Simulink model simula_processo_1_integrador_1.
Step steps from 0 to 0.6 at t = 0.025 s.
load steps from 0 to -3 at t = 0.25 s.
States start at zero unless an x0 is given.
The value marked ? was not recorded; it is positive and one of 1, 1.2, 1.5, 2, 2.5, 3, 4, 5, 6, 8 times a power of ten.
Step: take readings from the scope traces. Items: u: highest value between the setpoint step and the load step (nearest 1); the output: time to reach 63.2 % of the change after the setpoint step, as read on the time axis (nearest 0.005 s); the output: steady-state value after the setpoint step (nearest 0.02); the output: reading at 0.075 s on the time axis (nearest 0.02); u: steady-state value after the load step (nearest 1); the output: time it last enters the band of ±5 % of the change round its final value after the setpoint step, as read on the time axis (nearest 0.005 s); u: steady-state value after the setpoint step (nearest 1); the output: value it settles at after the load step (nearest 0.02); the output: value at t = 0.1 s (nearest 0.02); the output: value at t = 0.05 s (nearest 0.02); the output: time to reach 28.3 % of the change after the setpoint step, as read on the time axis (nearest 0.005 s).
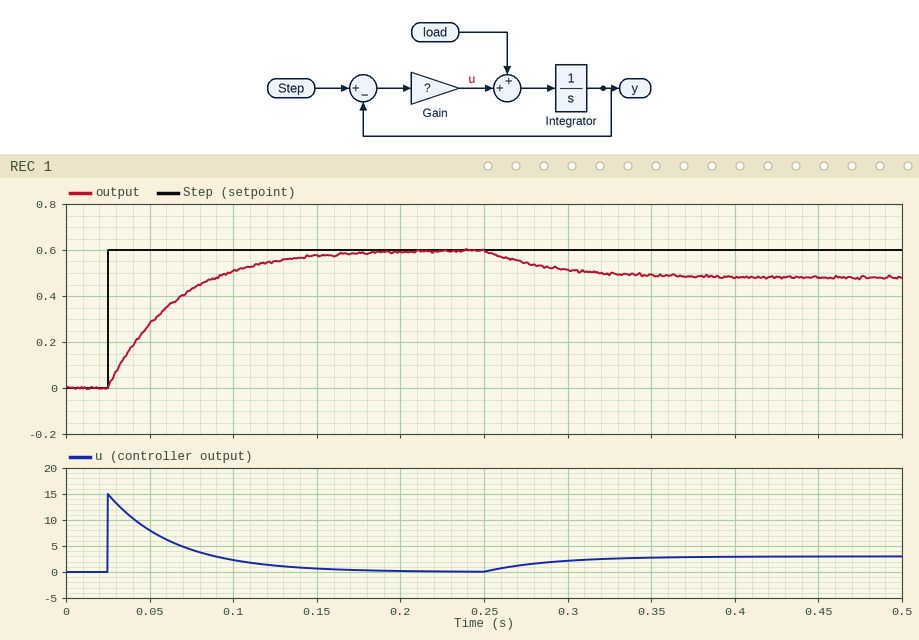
15
0.065 s
0.60
0.42
3
0.145 s
0
0.48
0.50
0.28
0.040 s
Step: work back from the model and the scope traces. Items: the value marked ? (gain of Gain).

25
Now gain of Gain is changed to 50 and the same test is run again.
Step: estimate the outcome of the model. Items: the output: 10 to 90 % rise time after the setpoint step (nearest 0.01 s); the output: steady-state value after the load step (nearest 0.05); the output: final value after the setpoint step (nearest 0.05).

0.04 s
0.55
0.60
